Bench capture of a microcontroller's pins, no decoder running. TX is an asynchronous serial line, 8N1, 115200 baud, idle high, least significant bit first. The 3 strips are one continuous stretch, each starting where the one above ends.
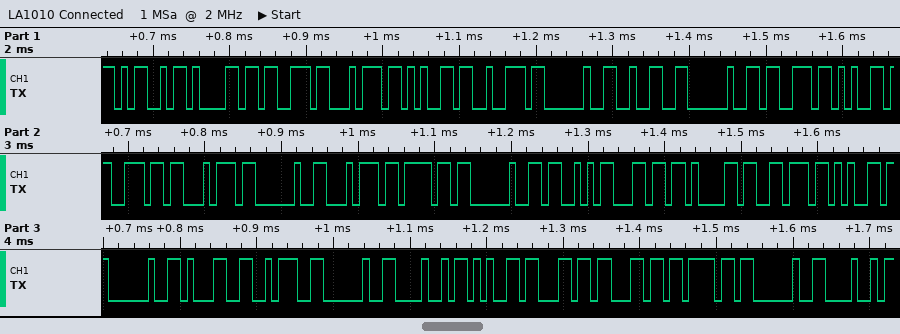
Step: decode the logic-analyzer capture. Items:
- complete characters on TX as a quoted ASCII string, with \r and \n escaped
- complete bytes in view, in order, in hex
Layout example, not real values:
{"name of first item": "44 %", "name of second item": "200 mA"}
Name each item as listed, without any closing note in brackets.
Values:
{"complete characters on TX as a quoted ASCII string, with \\r and \\n escaped": "\"Master 2 sent to Slave 1: Hello H\"", "complete bytes in view, in order, in hex": "0x4D 0x61 0x73 0x74 0x65 0x72 0x20 0x32 0x20 0x73 0x65 0x6E 0x74 0x20 0x74 0x6F 0x20 0x53 0x6C 0x61 0x76 0x65 0x20 0x31 0x3A 0x20 0x48 0x65 0x6C 0x6C 0x6F 0x20 0x48"}
